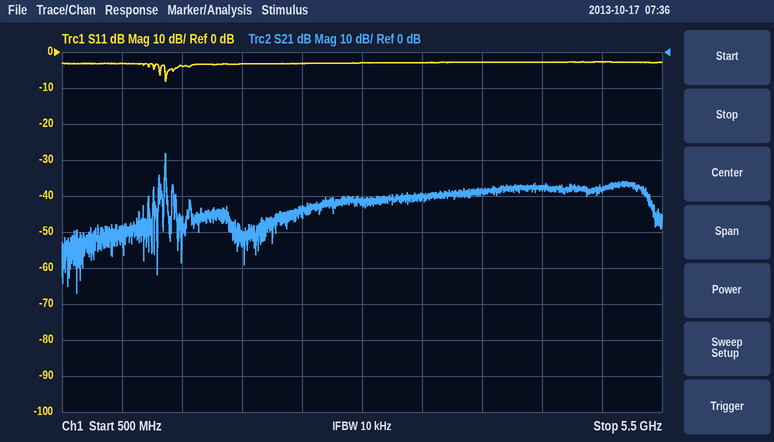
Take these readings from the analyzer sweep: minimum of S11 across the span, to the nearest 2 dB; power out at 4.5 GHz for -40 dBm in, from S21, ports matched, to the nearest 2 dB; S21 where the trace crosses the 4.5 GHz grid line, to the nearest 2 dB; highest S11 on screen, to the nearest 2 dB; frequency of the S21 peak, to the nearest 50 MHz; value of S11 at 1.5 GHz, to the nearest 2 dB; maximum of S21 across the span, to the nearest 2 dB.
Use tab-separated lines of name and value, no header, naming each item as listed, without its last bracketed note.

minimum of S11 across the span, to the nearest 2 dB	-8 dB
power out at 4.5 GHz for -40 dBm in, from S21, ports matched, to the nearest 2 dB	-78 dBm
S21 where the trace crosses the 4.5 GHz grid line, to the nearest 2 dB	-38 dB
highest S11 on screen, to the nearest 2 dB	-2 dB
frequency of the S21 peak, to the nearest 50 MHz	1.35 GHz
value of S11 at 1.5 GHz, to the nearest 2 dB	-4 dB
maximum of S21 across the span, to the nearest 2 dB	-28 dB
